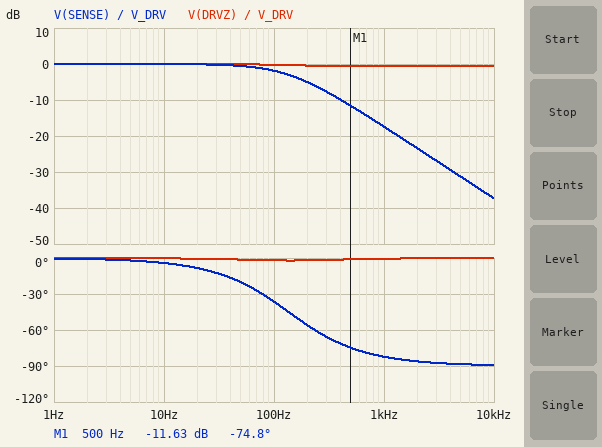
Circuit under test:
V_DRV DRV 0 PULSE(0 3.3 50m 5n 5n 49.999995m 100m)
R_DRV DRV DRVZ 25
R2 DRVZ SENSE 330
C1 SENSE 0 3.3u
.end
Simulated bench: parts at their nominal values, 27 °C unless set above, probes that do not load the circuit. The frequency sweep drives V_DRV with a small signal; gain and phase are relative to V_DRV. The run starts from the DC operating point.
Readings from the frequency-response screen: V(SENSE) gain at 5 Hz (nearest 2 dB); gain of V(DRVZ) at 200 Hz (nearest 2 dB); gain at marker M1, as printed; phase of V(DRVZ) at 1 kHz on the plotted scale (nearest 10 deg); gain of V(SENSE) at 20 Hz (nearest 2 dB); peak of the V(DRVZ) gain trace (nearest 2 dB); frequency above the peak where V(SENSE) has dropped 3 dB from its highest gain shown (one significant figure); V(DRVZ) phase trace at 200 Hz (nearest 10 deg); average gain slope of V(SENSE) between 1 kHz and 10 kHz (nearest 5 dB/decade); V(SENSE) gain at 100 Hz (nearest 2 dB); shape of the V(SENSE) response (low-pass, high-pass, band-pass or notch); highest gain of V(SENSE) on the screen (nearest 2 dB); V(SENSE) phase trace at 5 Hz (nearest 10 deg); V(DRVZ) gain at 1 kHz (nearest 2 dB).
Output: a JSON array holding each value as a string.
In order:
["0 dB", "0 dB", "-11.63 dB", "0 deg", "0 dB", "0 dB", "100 Hz", "0 deg", "-20 dB/decade", "-2 dB", "low-pass", "0 dB", "0 deg", "0 dB"]
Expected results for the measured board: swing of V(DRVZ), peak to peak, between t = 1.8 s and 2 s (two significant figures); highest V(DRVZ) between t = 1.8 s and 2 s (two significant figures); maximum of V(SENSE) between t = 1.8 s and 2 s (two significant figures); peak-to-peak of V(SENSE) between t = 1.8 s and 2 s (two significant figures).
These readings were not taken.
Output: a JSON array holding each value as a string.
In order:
["3.3 V", "3.3 V", "3.3 V", "3.3 V"]
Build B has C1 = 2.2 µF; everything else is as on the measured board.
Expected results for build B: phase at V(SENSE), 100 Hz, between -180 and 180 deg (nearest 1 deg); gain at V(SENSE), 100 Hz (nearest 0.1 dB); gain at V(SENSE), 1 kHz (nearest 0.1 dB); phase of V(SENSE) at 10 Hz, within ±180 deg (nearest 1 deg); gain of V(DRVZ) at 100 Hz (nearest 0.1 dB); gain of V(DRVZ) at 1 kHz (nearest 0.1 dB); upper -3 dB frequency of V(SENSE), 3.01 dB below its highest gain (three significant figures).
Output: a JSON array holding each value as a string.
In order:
["-26 deg", "-0.9 dB", "-14.0 dB", "-3 deg", "-0.1 dB", "-0.6 dB", "204 Hz"]
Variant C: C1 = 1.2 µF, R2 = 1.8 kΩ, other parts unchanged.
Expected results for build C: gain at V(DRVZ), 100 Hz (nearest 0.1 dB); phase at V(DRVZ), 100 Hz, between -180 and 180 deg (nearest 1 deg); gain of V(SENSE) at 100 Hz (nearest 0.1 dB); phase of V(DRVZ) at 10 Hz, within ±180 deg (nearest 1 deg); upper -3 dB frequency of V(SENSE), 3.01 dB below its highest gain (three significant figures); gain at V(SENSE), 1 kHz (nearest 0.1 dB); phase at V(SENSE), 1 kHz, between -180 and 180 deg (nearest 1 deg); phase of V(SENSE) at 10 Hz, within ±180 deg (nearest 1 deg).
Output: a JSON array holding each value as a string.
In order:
["-0.1 dB", "0 deg", "-4.6 dB", "0 deg", "72.7 Hz", "-22.8 dB", "-86 deg", "-8 deg"]
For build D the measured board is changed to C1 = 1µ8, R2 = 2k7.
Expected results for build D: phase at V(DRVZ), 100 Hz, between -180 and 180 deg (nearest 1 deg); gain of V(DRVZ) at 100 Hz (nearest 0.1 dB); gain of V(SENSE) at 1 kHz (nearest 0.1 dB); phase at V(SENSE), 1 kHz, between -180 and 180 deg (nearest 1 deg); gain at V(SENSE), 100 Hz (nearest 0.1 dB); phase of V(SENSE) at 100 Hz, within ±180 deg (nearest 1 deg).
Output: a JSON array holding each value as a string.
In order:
["0 deg", "-0.1 dB", "-29.8 dB", "-88 deg", "-10.2 dB", "-72 deg"]
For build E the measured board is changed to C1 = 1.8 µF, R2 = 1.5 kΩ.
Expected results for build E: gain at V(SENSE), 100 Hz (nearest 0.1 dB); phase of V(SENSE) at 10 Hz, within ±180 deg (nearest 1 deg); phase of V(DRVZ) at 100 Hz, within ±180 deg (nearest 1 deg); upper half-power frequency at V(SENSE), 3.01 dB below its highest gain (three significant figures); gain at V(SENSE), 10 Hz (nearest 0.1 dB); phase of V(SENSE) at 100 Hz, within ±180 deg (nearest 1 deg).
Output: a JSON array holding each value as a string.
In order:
["-6.0 dB", "-10 deg", "0 deg", "58.0 Hz", "-0.1 dB", "-60 deg"]
